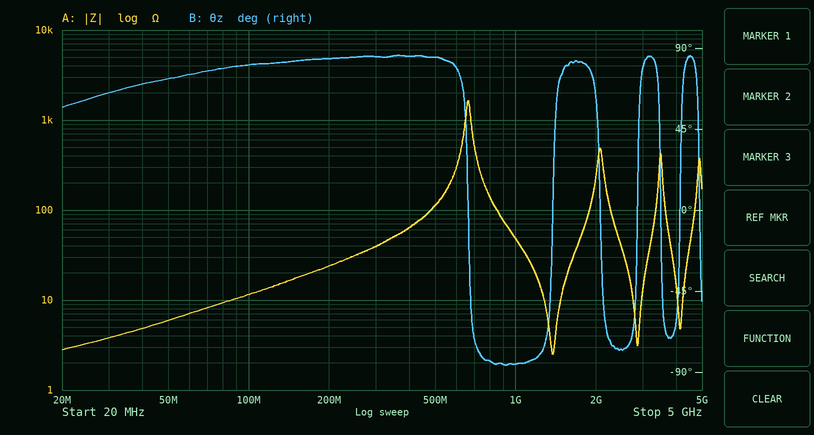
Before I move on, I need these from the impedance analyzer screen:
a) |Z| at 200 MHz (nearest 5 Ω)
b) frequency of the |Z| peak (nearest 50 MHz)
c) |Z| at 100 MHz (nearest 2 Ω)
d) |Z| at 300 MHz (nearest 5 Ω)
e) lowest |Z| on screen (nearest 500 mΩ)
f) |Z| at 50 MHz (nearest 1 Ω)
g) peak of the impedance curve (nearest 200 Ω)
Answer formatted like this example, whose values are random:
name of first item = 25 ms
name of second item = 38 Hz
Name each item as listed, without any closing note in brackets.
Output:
|Z| at 200 MHz = 25 Ω
frequency of the |Z| peak = 650 MHz
|Z| at 100 MHz = 12 Ω
|Z| at 300 MHz = 40 Ω
lowest |Z| on screen = 2.5 Ω
|Z| at 50 MHz = 6 Ω
peak of the impedance curve = 1.6 kΩ
